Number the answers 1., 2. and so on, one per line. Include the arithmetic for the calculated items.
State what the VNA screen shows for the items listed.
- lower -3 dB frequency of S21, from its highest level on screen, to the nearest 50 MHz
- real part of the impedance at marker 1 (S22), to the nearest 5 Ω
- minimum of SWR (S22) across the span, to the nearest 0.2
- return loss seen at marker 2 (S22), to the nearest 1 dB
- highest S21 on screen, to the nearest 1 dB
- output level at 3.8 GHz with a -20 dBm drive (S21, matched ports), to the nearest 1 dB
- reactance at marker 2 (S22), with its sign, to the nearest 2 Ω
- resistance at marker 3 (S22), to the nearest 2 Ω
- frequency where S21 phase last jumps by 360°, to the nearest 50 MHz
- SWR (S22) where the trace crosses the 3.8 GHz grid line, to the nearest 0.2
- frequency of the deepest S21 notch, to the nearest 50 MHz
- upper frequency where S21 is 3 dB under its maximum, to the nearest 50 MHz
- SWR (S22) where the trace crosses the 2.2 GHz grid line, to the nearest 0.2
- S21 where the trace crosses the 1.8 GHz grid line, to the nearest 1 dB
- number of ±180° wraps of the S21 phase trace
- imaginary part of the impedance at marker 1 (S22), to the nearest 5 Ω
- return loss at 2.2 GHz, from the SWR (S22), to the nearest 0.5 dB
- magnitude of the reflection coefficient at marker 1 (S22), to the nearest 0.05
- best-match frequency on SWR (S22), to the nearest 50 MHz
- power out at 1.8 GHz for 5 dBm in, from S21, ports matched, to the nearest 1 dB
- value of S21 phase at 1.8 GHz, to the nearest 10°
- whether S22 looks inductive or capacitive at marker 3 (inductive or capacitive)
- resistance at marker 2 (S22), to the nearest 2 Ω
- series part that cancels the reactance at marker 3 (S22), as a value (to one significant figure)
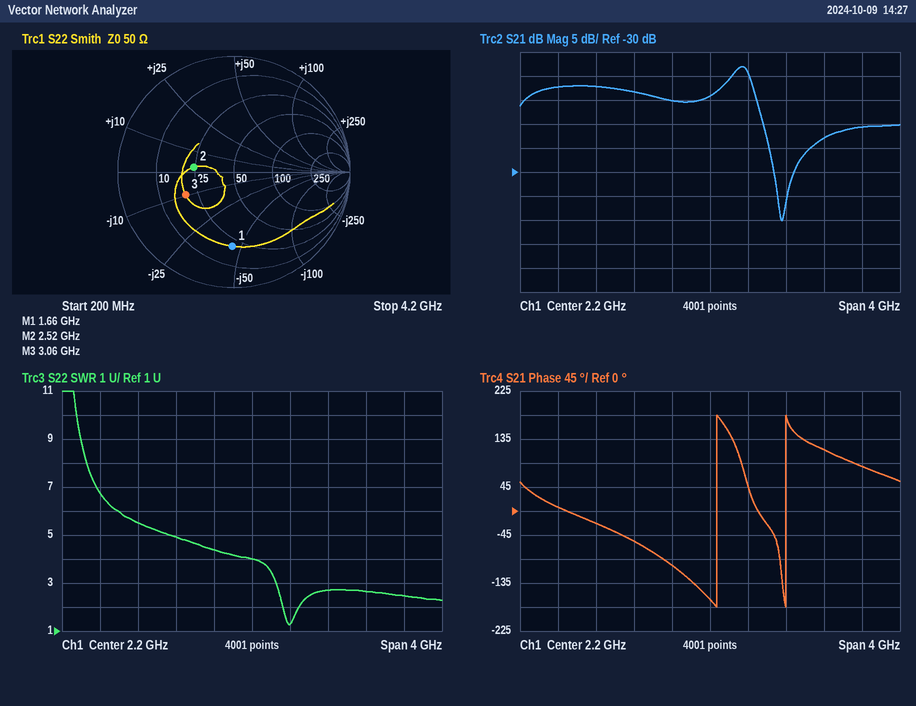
1. 2.40 GHz
2. 20 Ω
3. 1.2
4. 9 dB
5. -8 dB
6. -20 dBm + (-21 dB) = -41 dBm
7. +2 Ω
8. 20 Ω
9. 3.00 GHz
10. 2.4
11. 2.95 GHz
12. 2.65 GHz
13. 4.0
14. -15 dB
15. 2
16. -45 Ω
17. −20 log10((4 − 1)/(4 + 1)) ≈ 4.44 dB, so 4.5 dB to the nearest 0.5 dB
18. 0.65
19. 2.60 GHz
20. 5 dBm + (-15 dB) = -10 dBm
21. -100°
22. capacitive
23. 24 Ω
24. L = 10 Ω/(2π × 3.06 GHz) ≈ 520 pH, so 500 pH to one significant figure
